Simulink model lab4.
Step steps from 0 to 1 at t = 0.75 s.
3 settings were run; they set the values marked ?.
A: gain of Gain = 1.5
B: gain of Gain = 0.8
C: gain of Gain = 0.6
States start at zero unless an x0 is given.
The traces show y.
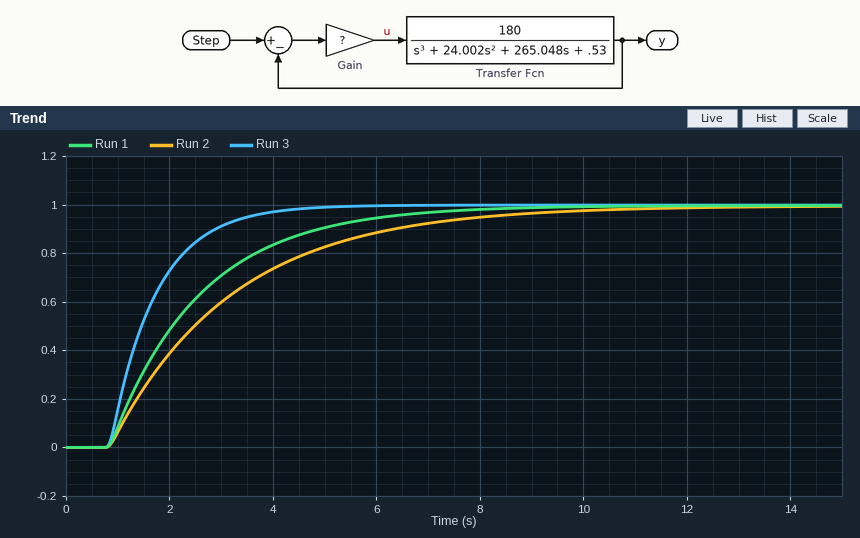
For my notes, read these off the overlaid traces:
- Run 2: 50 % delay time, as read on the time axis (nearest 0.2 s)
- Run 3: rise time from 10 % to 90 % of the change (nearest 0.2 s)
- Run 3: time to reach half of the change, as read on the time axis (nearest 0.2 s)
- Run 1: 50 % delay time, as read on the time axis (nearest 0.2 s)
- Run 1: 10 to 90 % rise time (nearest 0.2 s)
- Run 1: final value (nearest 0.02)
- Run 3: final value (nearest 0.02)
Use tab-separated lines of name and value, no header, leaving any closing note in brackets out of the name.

Run 2: 50 % delay time, as read on the time axis	2.4 s
Run 3: rise time from 10 % to 90 % of the change	2.0 s
Run 3: time to reach half of the change, as read on the time axis	1.4 s
Run 1: 50 % delay time, as read on the time axis	2.0 s
Run 1: 10 to 90 % rise time	3.8 s
Run 1: final value	1.00
Run 3: final value	1.00
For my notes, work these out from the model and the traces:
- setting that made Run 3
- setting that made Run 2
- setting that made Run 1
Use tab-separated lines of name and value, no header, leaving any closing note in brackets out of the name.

setting that made Run 3	A
setting that made Run 2	C
setting that made Run 1	B
